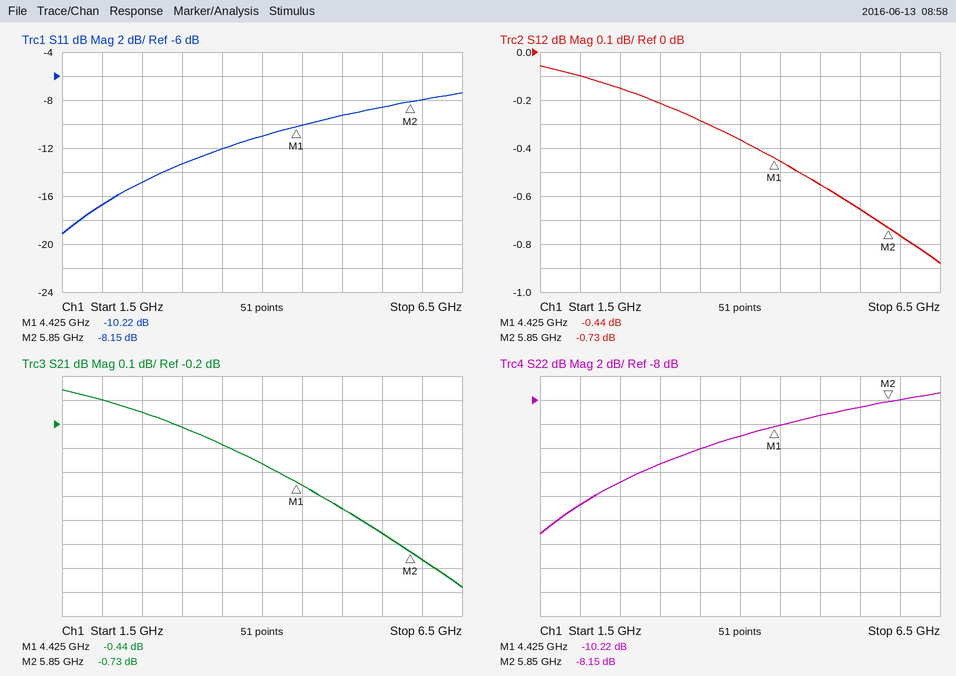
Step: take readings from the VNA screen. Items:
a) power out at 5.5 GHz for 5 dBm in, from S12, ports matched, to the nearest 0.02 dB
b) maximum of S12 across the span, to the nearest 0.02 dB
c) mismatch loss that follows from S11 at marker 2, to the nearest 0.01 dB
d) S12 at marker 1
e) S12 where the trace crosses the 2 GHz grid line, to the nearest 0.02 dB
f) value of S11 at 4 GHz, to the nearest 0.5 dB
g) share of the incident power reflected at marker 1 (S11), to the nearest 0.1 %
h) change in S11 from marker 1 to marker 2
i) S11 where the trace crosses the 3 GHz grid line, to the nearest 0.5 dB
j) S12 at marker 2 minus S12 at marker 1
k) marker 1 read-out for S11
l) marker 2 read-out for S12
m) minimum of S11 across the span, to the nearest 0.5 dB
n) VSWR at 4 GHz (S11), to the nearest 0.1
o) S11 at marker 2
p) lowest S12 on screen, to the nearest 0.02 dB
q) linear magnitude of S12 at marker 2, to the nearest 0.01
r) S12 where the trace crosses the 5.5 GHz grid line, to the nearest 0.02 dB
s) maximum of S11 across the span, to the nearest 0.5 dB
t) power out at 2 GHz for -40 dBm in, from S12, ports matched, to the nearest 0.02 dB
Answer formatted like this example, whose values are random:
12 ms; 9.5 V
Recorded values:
4.34 dBm; -0.06 dB; 0.72 dB; -0.44 dB; -0.10 dB; -11.0 dB; 9.5 %; 2.07 dB; -13.5 dB; -0.29 dB; -10.22 dB; -0.73 dB; -19.0 dB; 1.8; -8.15 dB; -0.88 dB; 0.92; -0.66 dB; -7.5 dB; -40.10 dBm
